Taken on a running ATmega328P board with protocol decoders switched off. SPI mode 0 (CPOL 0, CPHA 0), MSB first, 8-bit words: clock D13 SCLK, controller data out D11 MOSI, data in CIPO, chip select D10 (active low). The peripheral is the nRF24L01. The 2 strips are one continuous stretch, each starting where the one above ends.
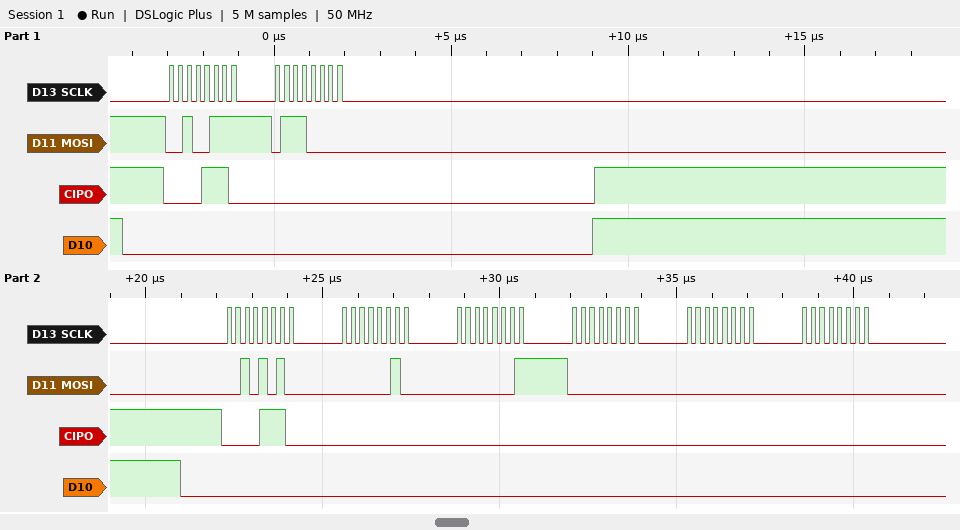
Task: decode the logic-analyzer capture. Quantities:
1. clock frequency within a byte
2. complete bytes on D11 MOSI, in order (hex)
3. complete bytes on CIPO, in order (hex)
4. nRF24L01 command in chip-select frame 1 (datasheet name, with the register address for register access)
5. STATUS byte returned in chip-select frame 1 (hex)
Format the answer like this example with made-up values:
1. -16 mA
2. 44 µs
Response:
1. 4 MHz
2. 27 70 2A 02 01 00 00 00
3. 0E 00 0E 00 00 00 00 00
4. W_REGISTER 0x07
5. 0x0E
